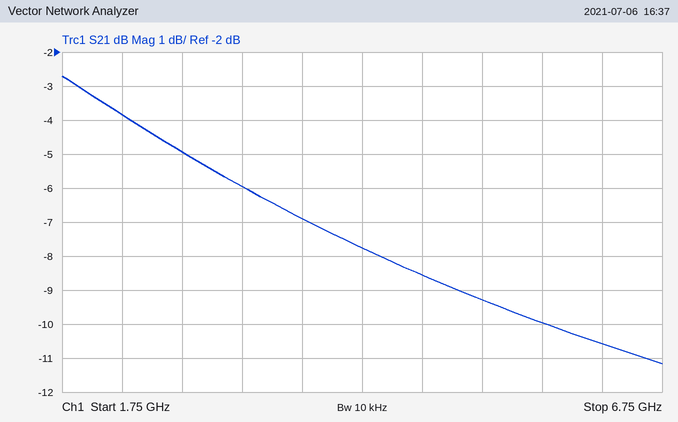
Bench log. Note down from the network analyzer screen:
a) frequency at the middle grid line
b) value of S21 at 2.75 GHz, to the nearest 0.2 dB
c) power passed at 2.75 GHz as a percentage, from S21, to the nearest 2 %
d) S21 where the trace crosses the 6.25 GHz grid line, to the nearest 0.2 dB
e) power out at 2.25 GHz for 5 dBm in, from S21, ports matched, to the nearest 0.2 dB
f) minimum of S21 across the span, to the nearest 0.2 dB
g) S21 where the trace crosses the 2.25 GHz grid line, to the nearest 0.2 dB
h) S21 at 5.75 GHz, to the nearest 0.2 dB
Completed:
4.25 GHz
-5.0 dB
32 %
-10.6 dB
1.2 dBm
-11.2 dB
-3.8 dB
-10.0 dB
